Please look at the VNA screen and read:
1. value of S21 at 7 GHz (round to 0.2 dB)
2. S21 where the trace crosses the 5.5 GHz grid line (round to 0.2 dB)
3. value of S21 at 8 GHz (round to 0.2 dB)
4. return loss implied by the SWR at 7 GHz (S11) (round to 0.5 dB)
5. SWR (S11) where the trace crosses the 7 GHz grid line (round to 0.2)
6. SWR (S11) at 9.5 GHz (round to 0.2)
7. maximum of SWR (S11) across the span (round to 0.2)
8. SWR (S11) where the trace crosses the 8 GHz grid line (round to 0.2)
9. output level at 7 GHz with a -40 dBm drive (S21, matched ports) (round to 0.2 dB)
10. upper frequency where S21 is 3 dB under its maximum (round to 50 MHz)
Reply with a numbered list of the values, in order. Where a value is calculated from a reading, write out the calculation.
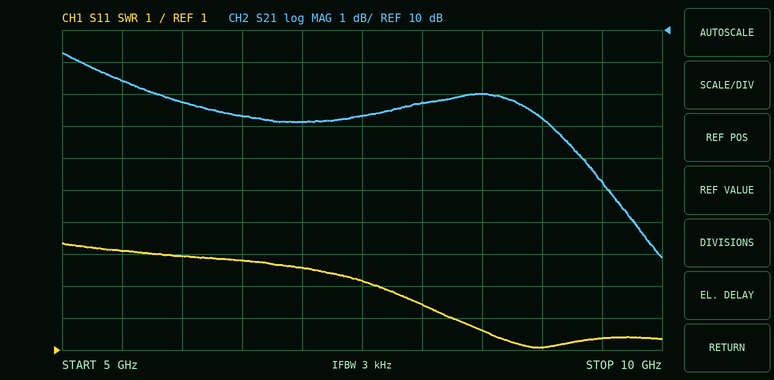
1. 7.2 dB
2. 8.4 dB
3. 7.8 dB
4. −20 log10((3.6 − 1)/(3.6 + 1)) ≈ 5.0 dB
5. 3.6
6. 1.4
7. 4.4
8. 2.4
9. -40 dBm + (7.2 dB) = -32.8 dBm
10. 9.25 GHz
